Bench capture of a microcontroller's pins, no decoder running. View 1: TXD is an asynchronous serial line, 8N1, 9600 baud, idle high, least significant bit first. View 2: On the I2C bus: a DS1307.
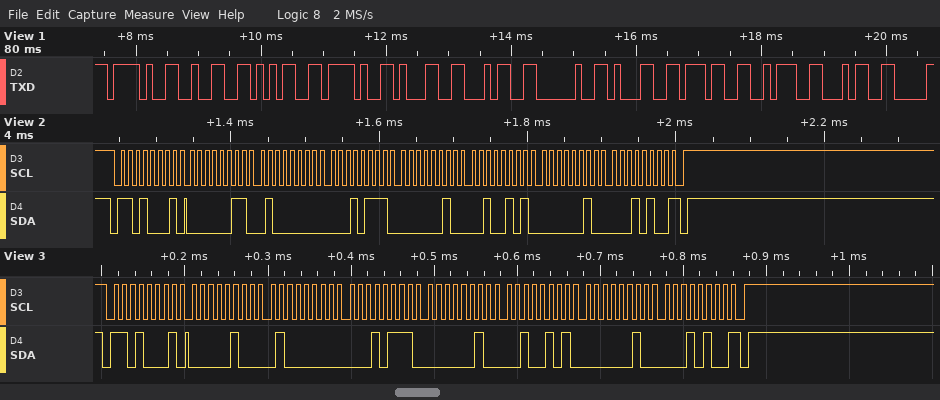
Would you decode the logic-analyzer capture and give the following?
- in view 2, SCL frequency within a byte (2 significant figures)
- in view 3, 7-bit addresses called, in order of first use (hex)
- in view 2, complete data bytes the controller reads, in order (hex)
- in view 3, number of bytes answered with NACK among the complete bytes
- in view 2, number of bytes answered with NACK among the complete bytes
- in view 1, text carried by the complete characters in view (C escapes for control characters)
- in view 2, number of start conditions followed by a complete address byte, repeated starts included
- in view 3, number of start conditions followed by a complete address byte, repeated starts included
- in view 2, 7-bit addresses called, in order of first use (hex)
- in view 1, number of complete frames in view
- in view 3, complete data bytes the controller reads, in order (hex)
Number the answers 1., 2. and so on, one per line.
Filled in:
1. 100 kHz
2. 0x68
3. 03 40 17 02 25 02 14
4. 1
5. 1
6. "/25/14 17:4"
7. 1
8. 1
9. 0x68
10. 11
11. 04 40 17 02 25 02 14
